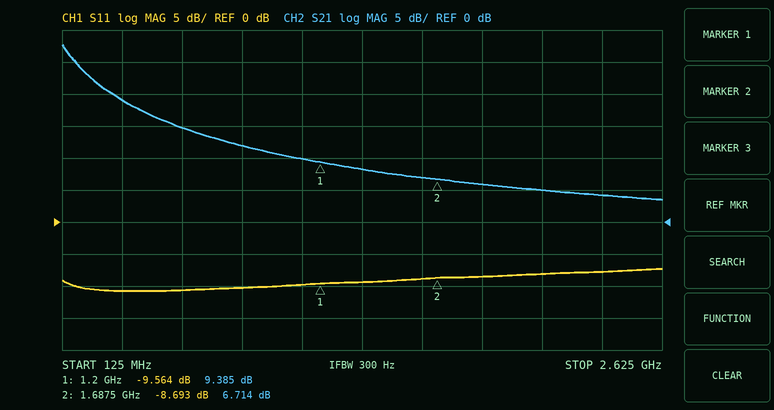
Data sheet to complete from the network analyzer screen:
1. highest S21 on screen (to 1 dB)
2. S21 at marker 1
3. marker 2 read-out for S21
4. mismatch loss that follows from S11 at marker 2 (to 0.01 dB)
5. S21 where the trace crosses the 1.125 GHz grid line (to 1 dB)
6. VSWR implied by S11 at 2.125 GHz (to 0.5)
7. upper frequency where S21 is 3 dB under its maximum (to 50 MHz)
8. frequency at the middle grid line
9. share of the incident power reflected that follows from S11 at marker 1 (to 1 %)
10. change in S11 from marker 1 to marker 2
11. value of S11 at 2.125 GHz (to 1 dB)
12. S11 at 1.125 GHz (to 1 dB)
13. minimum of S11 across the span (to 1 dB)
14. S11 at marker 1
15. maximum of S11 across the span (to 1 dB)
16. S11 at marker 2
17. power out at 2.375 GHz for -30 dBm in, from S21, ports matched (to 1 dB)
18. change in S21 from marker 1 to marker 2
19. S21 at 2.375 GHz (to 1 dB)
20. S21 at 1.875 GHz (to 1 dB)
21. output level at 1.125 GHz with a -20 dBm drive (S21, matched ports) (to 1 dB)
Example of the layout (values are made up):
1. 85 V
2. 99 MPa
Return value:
1. 28 dB
2. 9.385 dB
3. 6.714 dB
4. 0.63 dB
5. 10 dB
6. 2.5
7. 200 MHz
8. 1.375 GHz
9. 11 %
10. 0.871 dB
11. -8 dB
12. -10 dB
13. -11 dB
14. -9.564 dB
15. -7 dB
16. -8.693 dB
17. -26 dBm
18. -2.671 dB
19. 4 dB
20. 6 dB
21. -10 dBm
